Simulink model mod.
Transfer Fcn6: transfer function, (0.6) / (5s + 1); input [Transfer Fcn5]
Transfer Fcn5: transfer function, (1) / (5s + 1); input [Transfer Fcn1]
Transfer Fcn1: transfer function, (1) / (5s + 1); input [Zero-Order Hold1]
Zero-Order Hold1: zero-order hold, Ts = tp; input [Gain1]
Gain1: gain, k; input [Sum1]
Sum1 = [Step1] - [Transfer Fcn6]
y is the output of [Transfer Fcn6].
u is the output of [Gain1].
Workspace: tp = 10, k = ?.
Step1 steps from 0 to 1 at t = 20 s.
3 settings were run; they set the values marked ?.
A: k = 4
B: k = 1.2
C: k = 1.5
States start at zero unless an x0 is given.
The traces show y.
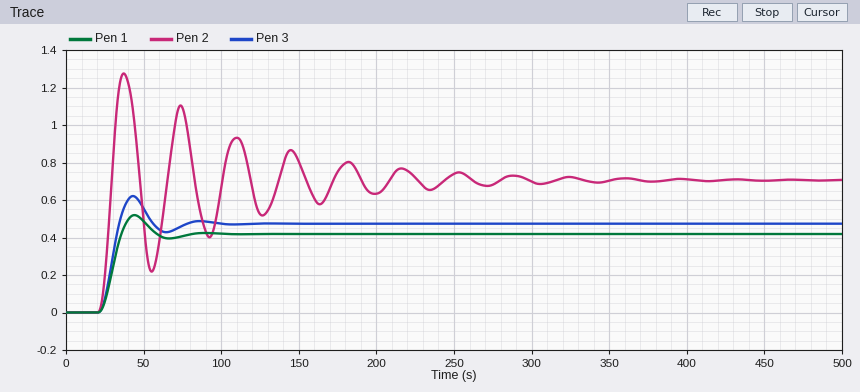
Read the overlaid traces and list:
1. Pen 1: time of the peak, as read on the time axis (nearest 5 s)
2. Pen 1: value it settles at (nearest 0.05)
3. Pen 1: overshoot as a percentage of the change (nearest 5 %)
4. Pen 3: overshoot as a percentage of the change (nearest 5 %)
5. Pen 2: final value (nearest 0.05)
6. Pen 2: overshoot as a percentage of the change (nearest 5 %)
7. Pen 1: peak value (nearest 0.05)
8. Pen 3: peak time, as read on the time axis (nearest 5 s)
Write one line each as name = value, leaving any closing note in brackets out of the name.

Pen 1: time of the peak, as read on the time axis = 45 s
Pen 1: value it settles at = 0.40
Pen 1: overshoot as a percentage of the change = 25 %
Pen 3: overshoot as a percentage of the change = 30 %
Pen 2: final value = 0.70
Pen 2: overshoot as a percentage of the change = 80 %
Pen 1: peak value = 0.50
Pen 3: peak time, as read on the time axis = 45 s
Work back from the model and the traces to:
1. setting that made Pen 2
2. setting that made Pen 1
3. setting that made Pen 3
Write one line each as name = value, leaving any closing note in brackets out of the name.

setting that made Pen 2 = A
setting that made Pen 1 = B
setting that made Pen 3 = C
